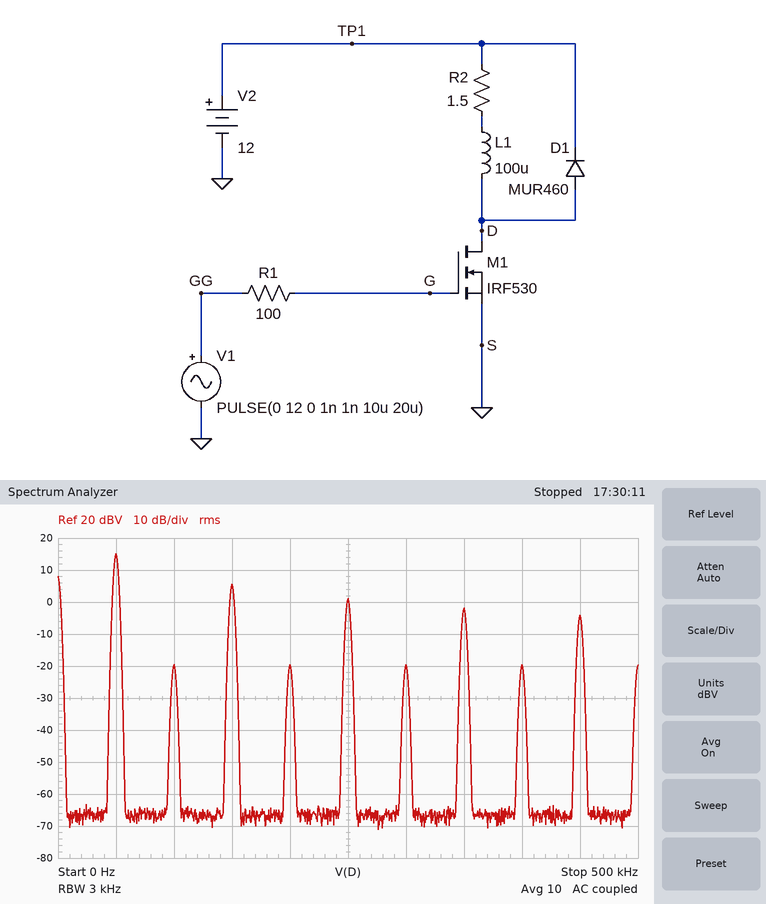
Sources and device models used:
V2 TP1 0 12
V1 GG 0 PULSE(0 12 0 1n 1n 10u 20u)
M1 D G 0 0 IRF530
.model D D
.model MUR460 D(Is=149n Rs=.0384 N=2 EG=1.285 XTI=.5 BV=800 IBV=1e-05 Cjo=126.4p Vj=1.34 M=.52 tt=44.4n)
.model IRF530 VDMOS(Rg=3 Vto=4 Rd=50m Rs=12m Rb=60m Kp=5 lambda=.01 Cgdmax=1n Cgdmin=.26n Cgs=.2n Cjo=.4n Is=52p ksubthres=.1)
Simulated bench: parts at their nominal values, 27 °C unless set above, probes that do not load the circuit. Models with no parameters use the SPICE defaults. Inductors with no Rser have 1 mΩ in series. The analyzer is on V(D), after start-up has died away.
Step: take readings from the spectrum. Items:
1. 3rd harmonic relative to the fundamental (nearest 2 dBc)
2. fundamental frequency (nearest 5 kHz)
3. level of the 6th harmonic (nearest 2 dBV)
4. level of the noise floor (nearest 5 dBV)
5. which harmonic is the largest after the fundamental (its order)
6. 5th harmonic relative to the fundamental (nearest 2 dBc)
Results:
-10 dBc
50 kHz
-20 dBV
-65 dBV
3
-14 dBc
